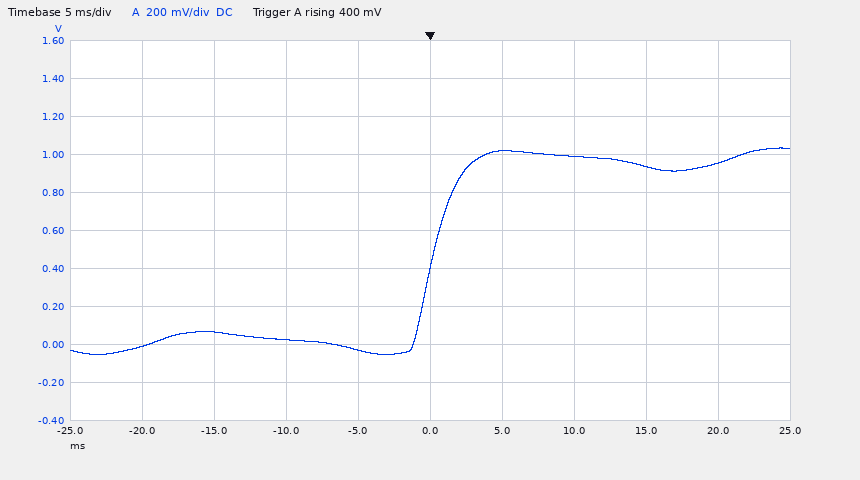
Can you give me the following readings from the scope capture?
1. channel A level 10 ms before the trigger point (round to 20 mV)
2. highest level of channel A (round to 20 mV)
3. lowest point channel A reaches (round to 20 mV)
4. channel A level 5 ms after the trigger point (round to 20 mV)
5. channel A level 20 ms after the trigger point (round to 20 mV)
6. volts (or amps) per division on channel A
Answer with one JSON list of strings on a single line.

["20 mV", "1.04 V", "-60 mV", "1.02 V", "960 mV", "200 mV"]
